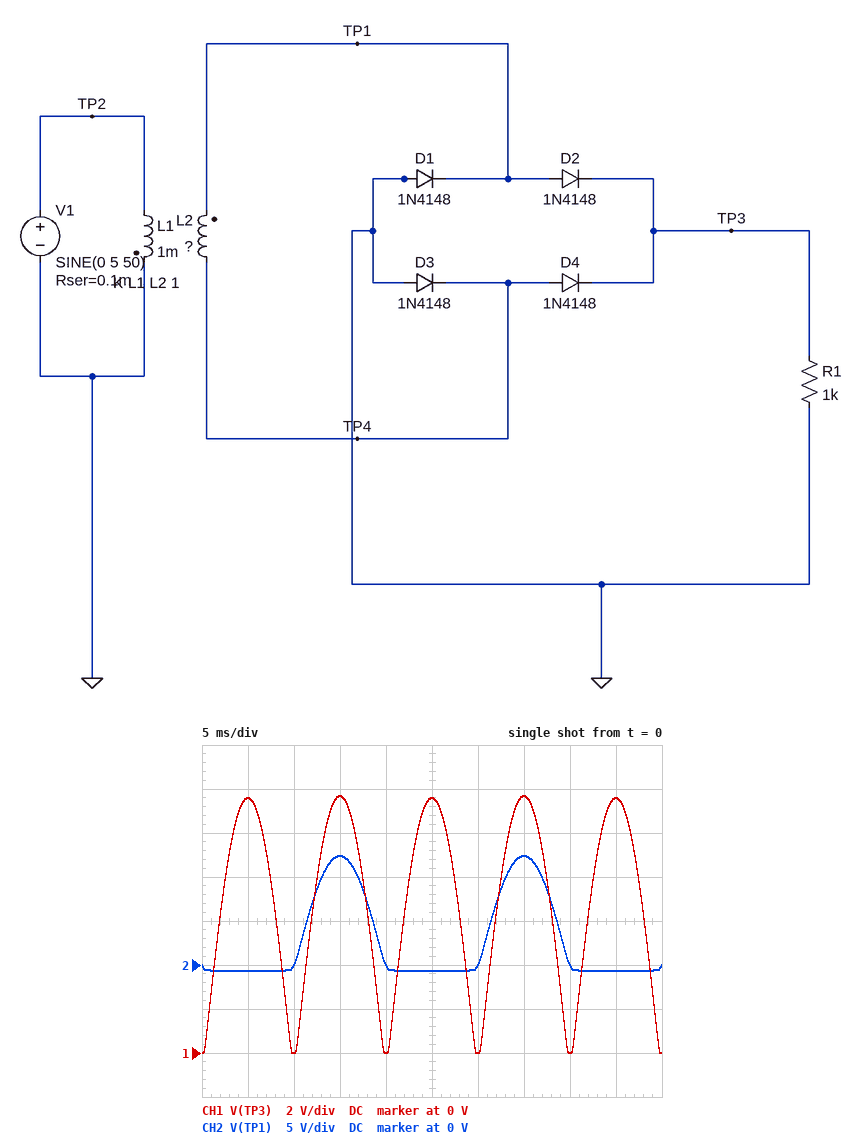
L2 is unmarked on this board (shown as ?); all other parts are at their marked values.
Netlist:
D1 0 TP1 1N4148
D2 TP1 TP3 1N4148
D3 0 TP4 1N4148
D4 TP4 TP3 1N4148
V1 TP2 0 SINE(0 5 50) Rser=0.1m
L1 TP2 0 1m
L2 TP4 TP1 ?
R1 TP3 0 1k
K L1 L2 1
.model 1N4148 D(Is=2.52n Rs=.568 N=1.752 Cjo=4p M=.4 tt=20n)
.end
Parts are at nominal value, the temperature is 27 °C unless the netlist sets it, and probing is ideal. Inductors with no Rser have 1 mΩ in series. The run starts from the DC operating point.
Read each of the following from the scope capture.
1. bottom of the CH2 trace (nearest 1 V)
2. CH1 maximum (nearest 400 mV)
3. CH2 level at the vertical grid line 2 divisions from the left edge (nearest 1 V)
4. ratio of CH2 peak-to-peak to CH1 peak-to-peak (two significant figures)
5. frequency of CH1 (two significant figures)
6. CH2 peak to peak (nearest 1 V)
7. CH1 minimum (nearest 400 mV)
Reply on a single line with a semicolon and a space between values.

-1 V; 11.6 V; 0 V; 1.1; 100 Hz; 13 V; 0 V
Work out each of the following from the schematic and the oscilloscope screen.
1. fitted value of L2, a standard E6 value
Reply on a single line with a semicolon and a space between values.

6.8 mH
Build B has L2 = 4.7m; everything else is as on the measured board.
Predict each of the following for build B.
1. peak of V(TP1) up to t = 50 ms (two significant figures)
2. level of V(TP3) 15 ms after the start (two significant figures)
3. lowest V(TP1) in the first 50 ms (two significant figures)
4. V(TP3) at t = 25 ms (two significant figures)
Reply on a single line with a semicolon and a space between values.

10 V; 9.5 V; -690 mV; 9.4 V
